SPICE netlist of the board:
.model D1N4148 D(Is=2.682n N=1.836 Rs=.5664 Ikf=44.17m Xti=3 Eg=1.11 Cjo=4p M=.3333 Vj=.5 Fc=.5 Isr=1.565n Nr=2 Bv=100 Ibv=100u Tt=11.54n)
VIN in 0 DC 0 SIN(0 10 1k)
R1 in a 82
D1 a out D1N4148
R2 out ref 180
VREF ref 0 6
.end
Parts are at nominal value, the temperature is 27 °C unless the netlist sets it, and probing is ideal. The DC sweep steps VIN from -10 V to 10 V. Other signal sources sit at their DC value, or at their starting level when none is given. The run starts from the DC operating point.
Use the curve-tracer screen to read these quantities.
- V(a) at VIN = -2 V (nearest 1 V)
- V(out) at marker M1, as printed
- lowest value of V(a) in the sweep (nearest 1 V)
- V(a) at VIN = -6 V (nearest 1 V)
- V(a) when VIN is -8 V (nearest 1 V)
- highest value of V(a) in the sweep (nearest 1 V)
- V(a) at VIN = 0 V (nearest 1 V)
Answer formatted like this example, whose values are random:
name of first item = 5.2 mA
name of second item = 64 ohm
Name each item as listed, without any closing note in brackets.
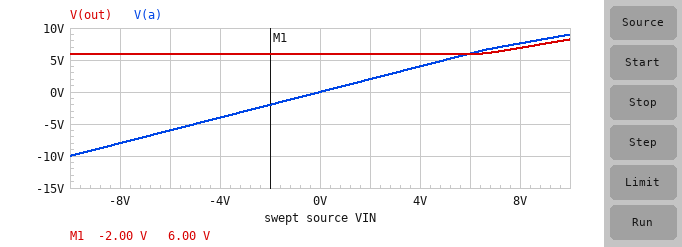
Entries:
V(a) at VIN = -2 V = -2 V
V(out) at marker M1, as printed = 6.00 V
lowest value of V(a) in the sweep = -10 V
V(a) at VIN = -6 V = -6 V
V(a) when VIN is -8 V = -8 V
highest value of V(a) in the sweep = 9 V
V(a) at VIN = 0 V = 0 V
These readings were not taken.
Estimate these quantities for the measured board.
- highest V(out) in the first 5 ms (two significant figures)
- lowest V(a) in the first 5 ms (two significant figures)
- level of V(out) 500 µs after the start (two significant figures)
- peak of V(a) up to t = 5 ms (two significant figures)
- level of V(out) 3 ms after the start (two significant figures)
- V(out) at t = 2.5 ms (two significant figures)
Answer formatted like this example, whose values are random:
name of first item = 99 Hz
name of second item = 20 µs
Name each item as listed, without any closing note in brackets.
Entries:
highest V(out) in the first 5 ms = 8.2 V
lowest V(a) in the first 5 ms = -10 V
level of V(out) 500 µs after the start = 6.0 V
peak of V(a) up to t = 5 ms = 9.0 V
level of V(out) 3 ms after the start = 6.0 V
V(out) at t = 2.5 ms = 6.0 V
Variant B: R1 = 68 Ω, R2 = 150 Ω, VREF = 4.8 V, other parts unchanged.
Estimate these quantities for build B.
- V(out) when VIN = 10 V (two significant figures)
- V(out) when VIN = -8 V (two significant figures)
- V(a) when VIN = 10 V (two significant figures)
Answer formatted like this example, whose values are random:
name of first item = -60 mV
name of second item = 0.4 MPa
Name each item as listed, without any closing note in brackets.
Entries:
V(out) when VIN = 10 V = 7.8 V
V(out) when VIN = -8 V = 4.8 V
V(a) when VIN = 10 V = 8.6 V
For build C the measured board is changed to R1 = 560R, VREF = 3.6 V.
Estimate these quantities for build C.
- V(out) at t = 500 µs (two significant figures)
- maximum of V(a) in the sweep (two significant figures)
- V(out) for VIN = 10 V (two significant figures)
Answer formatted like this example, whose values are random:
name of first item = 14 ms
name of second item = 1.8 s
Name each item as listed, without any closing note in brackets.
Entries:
V(out) at t = 500 µs = 3.6 V
maximum of V(a) in the sweep = 5.7 V
V(out) for VIN = 10 V = 5.0 V
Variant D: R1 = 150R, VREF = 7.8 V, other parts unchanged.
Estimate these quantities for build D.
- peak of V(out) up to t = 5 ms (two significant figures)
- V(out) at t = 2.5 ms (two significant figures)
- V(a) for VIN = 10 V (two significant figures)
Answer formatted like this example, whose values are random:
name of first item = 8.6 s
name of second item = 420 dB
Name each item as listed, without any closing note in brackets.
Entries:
peak of V(out) up to t = 5 ms = 8.6 V
V(out) at t = 2.5 ms = 7.8 V
V(a) for VIN = 10 V = 9.3 V
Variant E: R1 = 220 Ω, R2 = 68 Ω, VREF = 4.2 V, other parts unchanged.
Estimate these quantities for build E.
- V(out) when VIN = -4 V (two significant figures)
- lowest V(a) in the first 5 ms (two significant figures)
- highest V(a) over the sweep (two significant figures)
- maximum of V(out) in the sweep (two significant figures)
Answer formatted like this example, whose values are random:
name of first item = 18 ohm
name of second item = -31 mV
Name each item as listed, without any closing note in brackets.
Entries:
V(out) when VIN = -4 V = 4.2 V
lowest V(a) in the first 5 ms = -10 V
highest V(a) over the sweep = 6.2 V
maximum of V(out) in the sweep = 5.4 V
